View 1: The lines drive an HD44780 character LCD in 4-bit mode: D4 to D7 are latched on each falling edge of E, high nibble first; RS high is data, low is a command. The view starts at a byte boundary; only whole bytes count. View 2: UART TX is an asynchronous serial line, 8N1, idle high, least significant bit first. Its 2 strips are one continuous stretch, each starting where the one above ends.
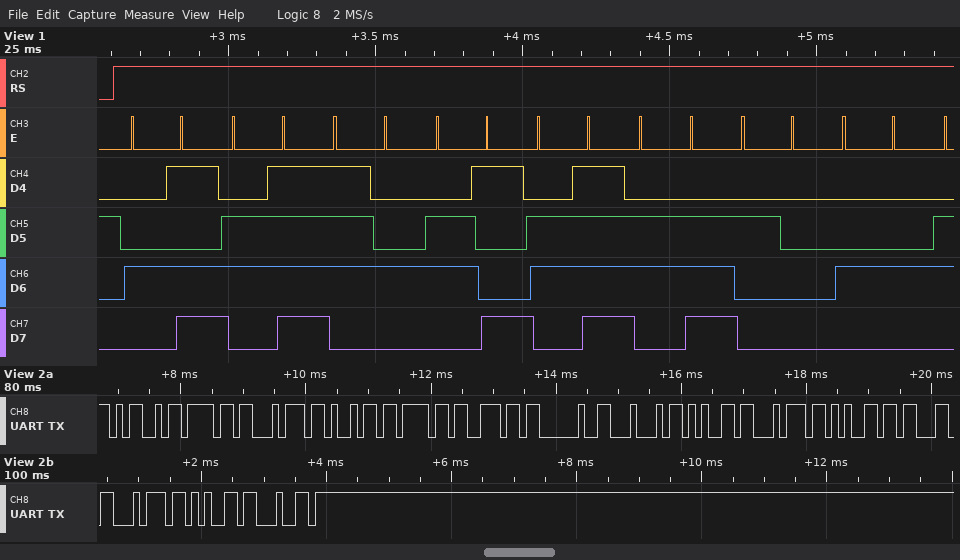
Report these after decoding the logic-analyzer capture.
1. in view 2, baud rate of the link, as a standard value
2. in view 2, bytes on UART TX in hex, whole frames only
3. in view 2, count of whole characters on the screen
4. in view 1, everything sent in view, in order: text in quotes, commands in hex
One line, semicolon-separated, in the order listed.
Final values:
9600 baud; 4D 6F 74 69 6F 6E 20 44 65 74 65 63 74 65 64; 15; "Motion D"
